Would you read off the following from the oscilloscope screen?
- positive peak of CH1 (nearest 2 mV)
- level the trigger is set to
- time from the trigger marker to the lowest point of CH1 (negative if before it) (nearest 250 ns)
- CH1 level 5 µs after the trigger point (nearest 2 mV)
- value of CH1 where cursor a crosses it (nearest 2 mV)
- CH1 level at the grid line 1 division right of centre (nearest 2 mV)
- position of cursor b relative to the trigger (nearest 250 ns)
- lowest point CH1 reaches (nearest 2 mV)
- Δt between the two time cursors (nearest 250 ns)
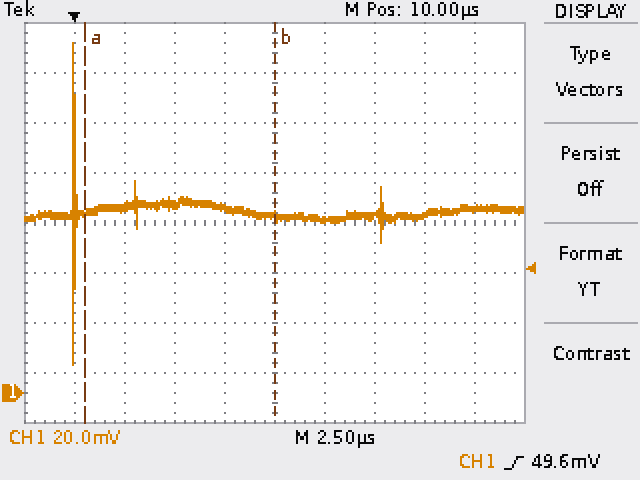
140 mV
49.6 mV
0.00 µs
76 mV
72 mV
70 mV
+10.00 µs
12 mV
9.50 µs
